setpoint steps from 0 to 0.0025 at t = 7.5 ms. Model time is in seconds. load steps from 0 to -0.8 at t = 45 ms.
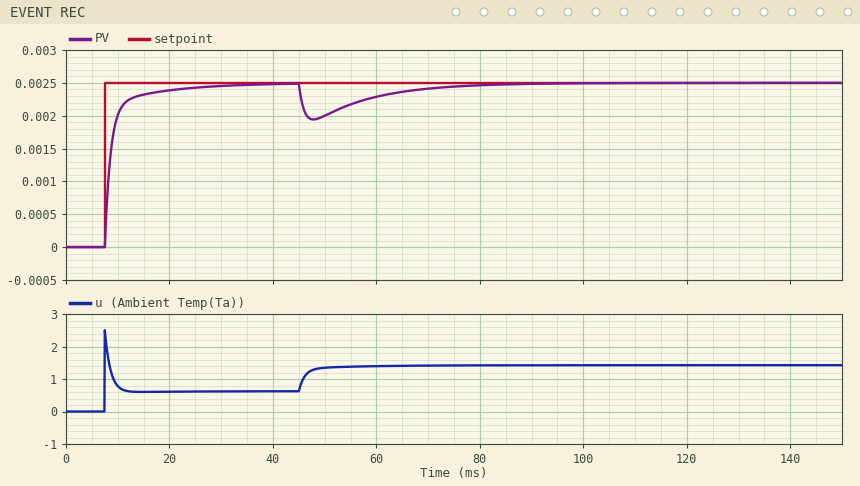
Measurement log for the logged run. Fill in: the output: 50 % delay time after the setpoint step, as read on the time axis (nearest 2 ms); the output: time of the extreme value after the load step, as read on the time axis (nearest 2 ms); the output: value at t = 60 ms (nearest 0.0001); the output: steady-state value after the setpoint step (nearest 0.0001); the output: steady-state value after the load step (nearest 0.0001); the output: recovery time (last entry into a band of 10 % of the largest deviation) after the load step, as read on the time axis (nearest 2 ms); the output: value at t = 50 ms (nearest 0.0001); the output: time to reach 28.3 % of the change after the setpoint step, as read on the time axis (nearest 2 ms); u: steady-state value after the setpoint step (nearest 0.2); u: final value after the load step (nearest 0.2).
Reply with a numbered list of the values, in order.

1. 8 ms
2. 48 ms
3. 0.0023
4. 0.0025
5. 0.0025
6. 76 ms
7. 0.0020
8. 8 ms
9. 0.6
10. 1.4
